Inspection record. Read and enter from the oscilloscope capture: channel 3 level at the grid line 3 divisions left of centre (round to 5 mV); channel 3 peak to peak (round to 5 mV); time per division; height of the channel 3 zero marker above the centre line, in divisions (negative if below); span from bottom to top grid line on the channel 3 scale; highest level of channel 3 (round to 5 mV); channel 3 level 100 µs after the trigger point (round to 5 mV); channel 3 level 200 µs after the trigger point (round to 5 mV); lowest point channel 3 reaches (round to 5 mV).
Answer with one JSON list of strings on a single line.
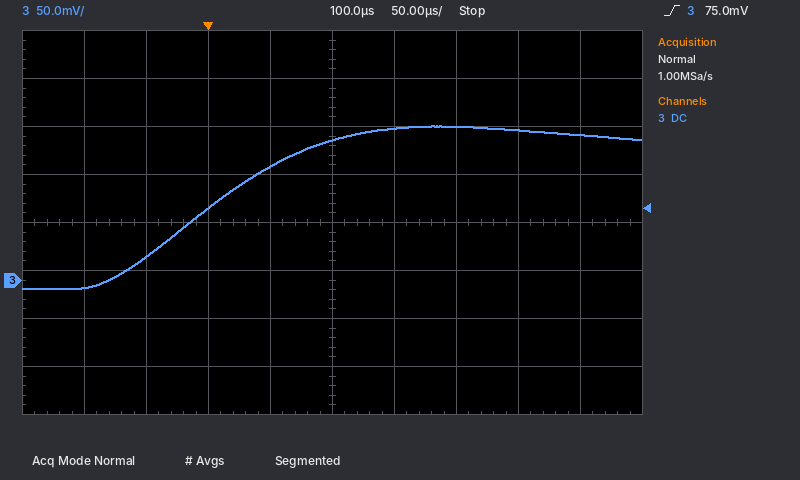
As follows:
["25 mV", "170 mV", "50 µs", "-1.2 div", "400 mV", "160 mV", "145 mV", "160 mV", "-10 mV"]
